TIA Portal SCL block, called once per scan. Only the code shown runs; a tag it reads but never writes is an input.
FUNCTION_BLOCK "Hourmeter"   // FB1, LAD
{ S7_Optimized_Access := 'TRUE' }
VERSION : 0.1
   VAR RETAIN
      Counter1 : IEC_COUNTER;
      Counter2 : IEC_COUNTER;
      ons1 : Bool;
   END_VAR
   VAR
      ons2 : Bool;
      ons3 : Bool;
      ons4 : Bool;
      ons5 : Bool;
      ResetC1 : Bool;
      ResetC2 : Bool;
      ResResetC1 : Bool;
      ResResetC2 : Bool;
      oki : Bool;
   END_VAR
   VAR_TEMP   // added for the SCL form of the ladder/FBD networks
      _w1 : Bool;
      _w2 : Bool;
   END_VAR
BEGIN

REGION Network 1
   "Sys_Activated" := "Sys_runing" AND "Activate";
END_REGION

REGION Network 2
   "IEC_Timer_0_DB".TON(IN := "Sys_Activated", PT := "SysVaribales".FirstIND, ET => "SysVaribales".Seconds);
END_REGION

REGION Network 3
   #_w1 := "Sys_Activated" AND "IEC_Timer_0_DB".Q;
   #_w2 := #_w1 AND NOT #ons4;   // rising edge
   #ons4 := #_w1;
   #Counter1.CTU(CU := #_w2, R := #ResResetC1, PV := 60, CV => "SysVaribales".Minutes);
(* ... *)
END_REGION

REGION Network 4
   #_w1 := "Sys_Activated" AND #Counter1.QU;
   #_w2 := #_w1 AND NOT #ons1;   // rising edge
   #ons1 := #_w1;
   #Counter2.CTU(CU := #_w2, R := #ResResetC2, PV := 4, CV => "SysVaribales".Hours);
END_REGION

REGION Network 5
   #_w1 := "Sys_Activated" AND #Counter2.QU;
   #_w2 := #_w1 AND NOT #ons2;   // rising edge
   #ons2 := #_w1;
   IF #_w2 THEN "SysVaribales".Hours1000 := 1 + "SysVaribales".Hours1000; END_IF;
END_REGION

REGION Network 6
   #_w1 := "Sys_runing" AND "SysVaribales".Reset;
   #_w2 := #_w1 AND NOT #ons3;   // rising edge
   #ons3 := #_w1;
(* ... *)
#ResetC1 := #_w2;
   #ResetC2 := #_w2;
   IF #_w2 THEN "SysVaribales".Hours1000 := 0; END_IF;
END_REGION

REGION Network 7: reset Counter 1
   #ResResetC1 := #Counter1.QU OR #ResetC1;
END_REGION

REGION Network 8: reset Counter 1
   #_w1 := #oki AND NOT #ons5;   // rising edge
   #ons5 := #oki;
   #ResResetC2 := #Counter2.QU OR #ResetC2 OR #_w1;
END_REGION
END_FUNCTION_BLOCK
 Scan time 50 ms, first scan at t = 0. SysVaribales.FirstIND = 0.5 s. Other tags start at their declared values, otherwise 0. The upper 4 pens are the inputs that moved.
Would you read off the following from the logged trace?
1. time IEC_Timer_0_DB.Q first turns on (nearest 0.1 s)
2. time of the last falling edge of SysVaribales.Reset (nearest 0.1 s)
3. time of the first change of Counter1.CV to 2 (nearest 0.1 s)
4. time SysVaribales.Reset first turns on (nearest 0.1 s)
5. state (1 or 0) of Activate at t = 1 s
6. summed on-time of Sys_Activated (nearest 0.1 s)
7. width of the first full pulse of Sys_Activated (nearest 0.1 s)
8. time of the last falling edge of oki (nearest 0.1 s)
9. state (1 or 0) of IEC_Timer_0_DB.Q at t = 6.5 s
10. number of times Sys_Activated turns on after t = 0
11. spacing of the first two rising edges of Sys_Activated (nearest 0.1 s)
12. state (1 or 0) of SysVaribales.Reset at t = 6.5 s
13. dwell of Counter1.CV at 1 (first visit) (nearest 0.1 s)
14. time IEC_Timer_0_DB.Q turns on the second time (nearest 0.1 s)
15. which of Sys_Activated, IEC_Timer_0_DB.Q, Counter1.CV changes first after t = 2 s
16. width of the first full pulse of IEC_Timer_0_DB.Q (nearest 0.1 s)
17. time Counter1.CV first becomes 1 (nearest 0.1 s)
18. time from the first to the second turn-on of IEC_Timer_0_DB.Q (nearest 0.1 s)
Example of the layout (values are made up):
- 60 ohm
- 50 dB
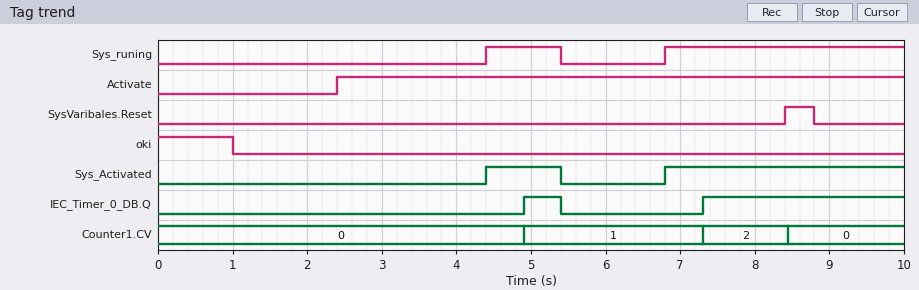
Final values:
- 4.9 s
- 8.8 s
- 7.3 s
- 8.4 s
- 0
- 4.2 s
- 1.0 s
- 1.0 s
- 0
- 2
- 2.4 s
- 0
- 2.4 s
- 7.3 s
- Sys_Activated
- 0.5 s
- 4.9 s
- 2.4 s
